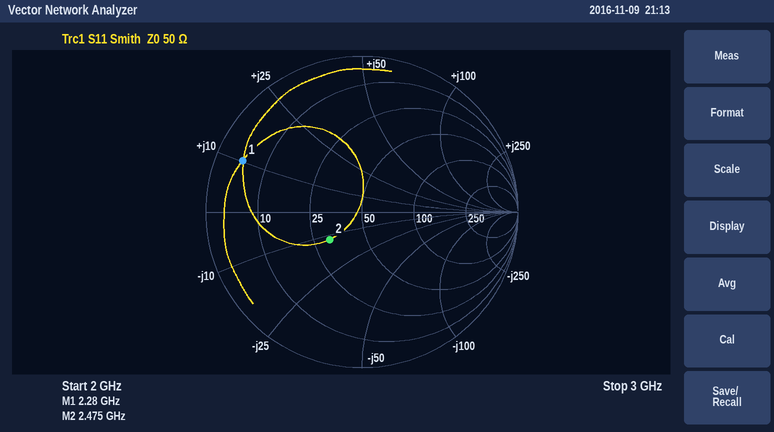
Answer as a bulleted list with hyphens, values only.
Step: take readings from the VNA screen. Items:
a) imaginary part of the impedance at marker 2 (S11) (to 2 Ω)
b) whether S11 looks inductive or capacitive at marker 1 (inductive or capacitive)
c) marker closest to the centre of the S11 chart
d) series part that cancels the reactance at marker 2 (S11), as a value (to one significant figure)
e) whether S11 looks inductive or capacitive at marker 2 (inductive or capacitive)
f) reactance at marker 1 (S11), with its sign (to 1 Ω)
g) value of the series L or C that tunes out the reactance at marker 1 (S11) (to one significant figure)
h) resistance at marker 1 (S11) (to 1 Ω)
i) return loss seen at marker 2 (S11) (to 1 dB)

- -12 Ω
- inductive
- marker 2
- 800 pH
- capacitive
- +10 Ω
- 7 pF
- 5 Ω
- 11 dB
